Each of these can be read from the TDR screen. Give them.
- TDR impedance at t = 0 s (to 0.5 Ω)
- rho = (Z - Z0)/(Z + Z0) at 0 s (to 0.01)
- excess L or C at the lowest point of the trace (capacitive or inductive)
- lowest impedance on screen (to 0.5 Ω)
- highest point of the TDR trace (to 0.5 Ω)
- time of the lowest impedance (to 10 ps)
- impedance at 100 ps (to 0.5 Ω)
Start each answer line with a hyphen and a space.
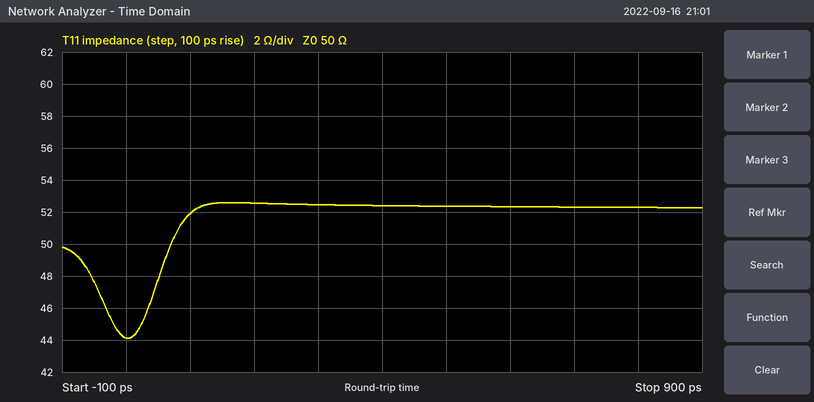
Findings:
- 44.0 Ω
- -0.06
- capacitive
- 44.0 Ω
- 52.5 Ω
- 0 ps
- 52.0 Ω
